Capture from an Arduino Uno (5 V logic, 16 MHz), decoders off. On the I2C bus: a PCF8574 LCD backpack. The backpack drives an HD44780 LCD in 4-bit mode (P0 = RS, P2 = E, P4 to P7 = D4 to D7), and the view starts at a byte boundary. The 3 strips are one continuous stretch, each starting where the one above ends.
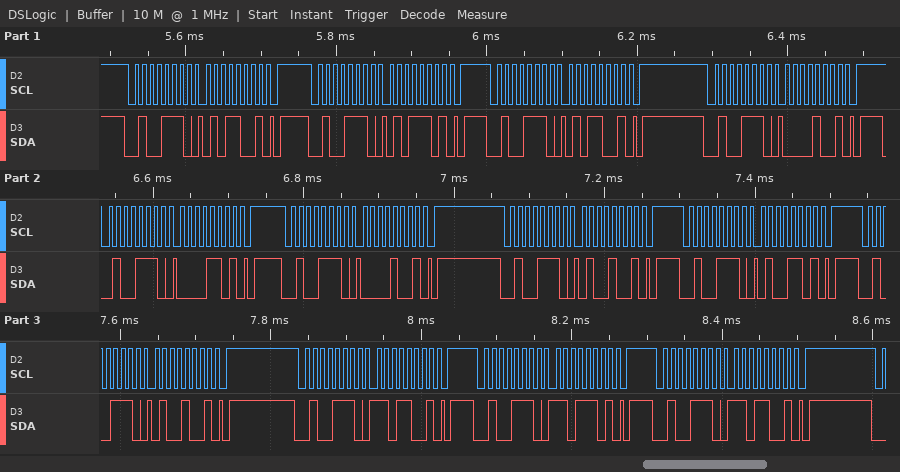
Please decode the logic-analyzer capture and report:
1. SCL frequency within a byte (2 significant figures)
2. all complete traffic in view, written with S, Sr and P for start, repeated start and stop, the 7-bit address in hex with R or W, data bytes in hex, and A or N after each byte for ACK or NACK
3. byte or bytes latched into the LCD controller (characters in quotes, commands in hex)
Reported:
100 kHz
S 27W A 59 A P S 27W A 5D A P S 27W A 59 A P S 27W A 09 A P S 27W A 0D A P S 27W A 09 A P S 27W A 49 A P S 27W A 4D A P S 27W A 49 A P S 27W A D9 A P S 27W A DD A P S 27W A D9 A P
'P' 'M'
